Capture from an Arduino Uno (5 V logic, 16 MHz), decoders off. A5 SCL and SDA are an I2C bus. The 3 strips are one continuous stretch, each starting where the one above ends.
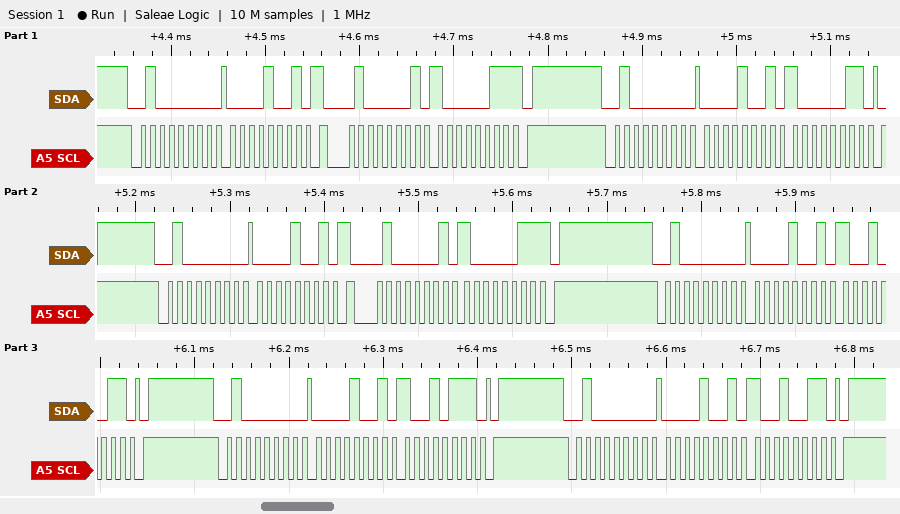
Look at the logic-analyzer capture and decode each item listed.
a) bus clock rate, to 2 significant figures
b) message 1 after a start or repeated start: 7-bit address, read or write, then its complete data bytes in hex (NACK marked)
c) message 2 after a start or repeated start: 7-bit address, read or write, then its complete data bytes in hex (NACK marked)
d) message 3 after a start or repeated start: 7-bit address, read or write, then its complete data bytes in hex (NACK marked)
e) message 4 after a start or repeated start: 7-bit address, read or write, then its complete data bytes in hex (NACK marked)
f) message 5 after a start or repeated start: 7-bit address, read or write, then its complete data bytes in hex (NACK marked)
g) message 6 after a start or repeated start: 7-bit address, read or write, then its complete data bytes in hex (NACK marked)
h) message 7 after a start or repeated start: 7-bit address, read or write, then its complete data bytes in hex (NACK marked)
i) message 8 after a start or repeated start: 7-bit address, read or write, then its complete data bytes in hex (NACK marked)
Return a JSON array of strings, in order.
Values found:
["100 kHz", "0x20 write: 09", "0x20 read: 83 NACK", "0x20 write: 09 83", "0x20 write: 09", "0x20 read: 83 NACK", "0x20 write: 09 93", "0x20 write: 09 97", "0x20 write: 09 93"]
